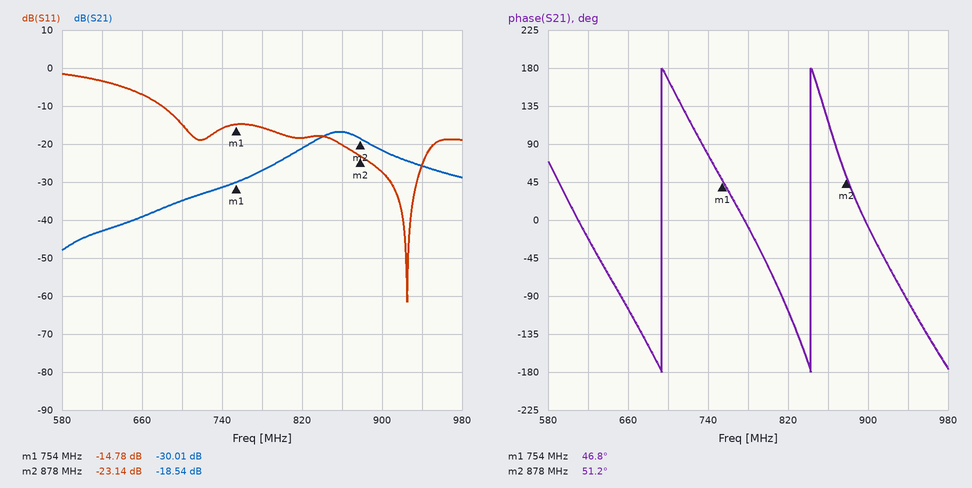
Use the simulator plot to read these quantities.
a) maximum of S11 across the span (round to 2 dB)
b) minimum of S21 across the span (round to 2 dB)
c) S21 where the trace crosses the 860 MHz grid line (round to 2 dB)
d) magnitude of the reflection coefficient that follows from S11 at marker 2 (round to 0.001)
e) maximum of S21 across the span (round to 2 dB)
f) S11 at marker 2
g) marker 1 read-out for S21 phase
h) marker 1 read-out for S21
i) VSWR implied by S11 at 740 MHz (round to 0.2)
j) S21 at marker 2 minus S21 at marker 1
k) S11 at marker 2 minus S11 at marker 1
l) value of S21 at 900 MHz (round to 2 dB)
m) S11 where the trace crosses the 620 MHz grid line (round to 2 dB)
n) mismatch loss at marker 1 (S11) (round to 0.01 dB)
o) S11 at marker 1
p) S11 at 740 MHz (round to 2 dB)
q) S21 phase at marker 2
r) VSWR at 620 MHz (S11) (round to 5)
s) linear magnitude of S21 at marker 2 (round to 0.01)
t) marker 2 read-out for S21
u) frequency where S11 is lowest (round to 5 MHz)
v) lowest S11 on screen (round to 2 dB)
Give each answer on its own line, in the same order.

-2 dB
-48 dB
-16 dB
0.070
-16 dB
-23.14 dB
46.8°
-30.01 dB
1.4
11.47 dB
-8.36 dB
-22 dB
-4 dB
0.15 dB
-14.78 dB
-16 dB
51.2°
5
0.12
-18.54 dB
925 MHz
-62 dB
